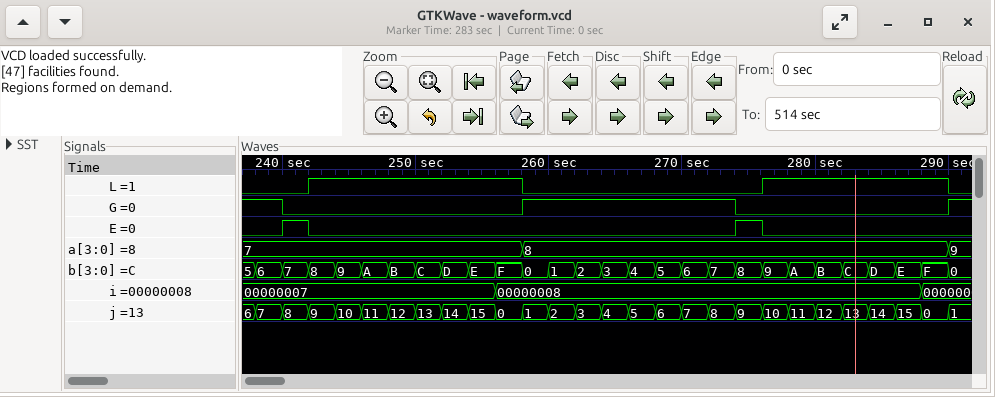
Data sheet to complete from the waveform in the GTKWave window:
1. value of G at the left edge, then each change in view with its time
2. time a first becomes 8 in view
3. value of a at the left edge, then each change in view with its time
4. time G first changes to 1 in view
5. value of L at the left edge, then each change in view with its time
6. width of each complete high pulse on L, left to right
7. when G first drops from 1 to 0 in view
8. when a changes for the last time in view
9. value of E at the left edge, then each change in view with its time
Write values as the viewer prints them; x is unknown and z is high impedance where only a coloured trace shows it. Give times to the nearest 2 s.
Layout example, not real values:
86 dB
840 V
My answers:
1, 0 at 240 s, 1 at 258 s, 0 at 274 s, 1 at 290 s
258 s
7, 8 at 258 s, 9 at 290 s
258 s
0, 1 at 242 s, 0 at 258 s, 1 at 276 s, 0 at 290 s
16 s, 14 s
240 s
290 s
0, 1 at 240 s, 0 at 242 s, 1 at 274 s, 0 at 276 s
